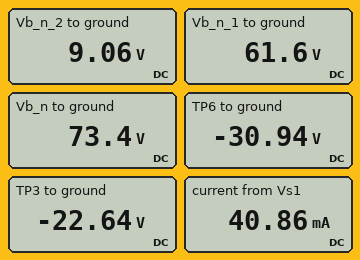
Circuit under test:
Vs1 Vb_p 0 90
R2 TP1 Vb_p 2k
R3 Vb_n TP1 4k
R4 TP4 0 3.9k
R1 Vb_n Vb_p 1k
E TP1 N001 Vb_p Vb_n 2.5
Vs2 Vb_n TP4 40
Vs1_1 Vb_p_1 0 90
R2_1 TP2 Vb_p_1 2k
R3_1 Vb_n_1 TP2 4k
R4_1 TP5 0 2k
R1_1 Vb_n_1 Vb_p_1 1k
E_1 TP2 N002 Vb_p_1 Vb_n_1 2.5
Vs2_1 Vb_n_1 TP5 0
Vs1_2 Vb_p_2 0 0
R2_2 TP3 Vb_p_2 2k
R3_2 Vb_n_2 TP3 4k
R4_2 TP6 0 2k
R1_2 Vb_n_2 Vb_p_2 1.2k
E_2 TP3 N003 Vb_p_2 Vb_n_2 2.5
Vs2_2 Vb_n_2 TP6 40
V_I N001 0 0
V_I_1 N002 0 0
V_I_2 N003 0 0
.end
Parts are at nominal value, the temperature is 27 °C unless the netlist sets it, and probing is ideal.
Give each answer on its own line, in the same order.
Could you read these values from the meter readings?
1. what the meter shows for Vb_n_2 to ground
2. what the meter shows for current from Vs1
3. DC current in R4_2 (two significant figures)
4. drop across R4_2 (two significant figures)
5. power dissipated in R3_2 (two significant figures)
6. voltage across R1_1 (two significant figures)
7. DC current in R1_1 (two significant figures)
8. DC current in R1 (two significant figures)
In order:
9.06 V
40.86 mA
15 mA
31 V
250 mW
28 V
28 mA
17 mA
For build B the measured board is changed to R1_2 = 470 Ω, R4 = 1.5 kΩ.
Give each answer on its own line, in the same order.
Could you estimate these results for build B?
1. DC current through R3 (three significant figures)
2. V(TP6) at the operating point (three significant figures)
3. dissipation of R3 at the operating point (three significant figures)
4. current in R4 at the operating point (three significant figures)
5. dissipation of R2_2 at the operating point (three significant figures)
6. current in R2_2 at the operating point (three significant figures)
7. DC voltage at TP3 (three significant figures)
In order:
3.28 mA
-34.3 V
43.0 mW
18.7 mA
102 mW
7.14 mA
-14.3 V
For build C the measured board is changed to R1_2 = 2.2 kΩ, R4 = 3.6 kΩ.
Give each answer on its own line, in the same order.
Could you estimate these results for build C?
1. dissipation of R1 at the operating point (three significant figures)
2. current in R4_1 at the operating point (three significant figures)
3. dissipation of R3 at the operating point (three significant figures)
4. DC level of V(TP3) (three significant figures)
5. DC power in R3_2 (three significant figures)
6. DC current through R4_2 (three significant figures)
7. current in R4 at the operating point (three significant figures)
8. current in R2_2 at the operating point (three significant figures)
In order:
286 mW
30.8 mA
238 mW
-27.3 V
366 mW
14.5 mA
9.19 mA
13.7 mA
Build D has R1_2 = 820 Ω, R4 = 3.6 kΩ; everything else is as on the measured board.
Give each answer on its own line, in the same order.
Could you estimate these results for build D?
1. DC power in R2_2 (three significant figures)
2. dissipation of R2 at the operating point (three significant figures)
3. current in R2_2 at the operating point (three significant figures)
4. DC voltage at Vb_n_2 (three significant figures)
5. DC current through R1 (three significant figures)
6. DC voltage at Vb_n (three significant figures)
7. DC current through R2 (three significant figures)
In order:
186 mW
1.14 W
9.64 mA
7.71 V
16.9 mA
73.1 V
23.9 mA
